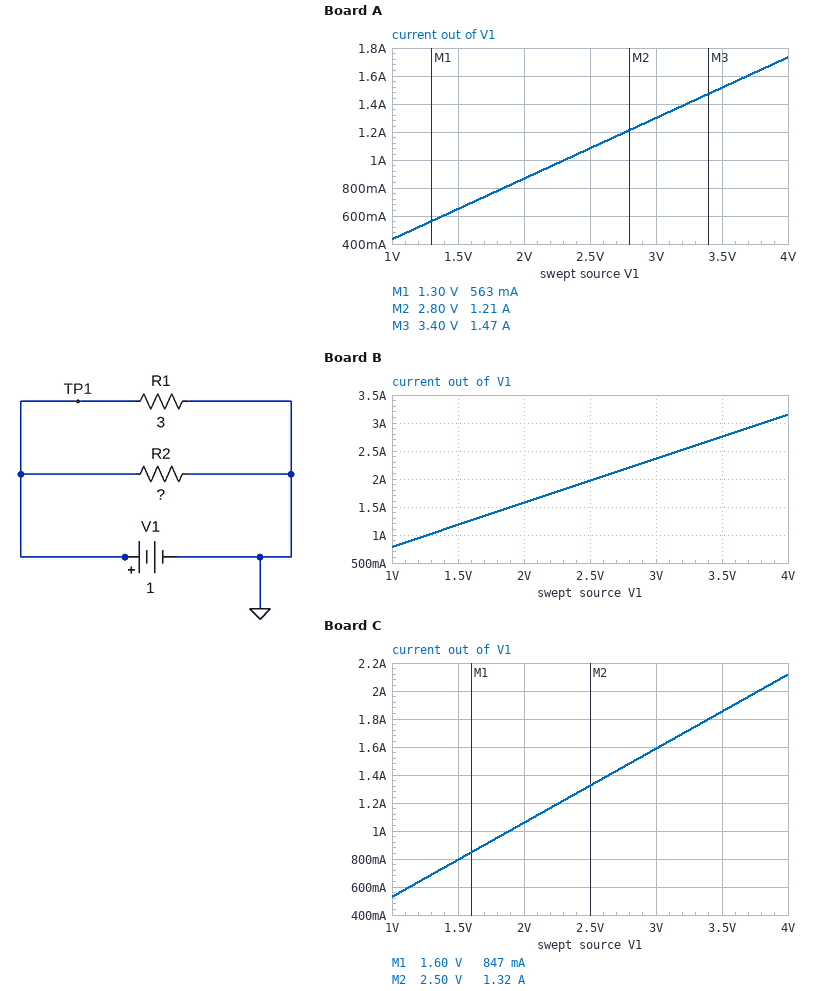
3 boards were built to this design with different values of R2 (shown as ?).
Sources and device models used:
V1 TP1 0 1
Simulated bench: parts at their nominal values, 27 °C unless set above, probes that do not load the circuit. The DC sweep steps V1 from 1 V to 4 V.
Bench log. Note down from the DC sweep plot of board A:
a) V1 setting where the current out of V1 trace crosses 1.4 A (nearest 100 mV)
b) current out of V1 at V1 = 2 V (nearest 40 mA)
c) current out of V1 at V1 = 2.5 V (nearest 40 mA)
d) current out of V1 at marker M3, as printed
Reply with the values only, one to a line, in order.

3.2 V
880 mA
1.08 A
1.47 A
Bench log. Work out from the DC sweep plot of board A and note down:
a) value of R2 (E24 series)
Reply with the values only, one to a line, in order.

10 Ω
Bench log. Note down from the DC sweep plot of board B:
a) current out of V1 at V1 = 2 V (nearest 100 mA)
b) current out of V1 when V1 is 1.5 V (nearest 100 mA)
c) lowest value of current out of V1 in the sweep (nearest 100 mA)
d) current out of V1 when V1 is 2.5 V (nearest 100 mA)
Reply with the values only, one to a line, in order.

1.6 A
1.2 A
800 mA
2.0 A
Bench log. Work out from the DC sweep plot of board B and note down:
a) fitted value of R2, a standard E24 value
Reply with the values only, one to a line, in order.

2.2 Ω
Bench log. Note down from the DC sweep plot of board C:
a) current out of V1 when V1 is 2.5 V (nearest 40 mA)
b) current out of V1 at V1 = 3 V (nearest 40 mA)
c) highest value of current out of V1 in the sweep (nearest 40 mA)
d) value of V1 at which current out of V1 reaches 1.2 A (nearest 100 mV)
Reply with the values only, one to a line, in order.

1.32 A
1.60 A
2.12 A
2.3 V
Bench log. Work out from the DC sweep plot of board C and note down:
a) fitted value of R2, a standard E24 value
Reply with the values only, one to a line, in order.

5.1 Ω
